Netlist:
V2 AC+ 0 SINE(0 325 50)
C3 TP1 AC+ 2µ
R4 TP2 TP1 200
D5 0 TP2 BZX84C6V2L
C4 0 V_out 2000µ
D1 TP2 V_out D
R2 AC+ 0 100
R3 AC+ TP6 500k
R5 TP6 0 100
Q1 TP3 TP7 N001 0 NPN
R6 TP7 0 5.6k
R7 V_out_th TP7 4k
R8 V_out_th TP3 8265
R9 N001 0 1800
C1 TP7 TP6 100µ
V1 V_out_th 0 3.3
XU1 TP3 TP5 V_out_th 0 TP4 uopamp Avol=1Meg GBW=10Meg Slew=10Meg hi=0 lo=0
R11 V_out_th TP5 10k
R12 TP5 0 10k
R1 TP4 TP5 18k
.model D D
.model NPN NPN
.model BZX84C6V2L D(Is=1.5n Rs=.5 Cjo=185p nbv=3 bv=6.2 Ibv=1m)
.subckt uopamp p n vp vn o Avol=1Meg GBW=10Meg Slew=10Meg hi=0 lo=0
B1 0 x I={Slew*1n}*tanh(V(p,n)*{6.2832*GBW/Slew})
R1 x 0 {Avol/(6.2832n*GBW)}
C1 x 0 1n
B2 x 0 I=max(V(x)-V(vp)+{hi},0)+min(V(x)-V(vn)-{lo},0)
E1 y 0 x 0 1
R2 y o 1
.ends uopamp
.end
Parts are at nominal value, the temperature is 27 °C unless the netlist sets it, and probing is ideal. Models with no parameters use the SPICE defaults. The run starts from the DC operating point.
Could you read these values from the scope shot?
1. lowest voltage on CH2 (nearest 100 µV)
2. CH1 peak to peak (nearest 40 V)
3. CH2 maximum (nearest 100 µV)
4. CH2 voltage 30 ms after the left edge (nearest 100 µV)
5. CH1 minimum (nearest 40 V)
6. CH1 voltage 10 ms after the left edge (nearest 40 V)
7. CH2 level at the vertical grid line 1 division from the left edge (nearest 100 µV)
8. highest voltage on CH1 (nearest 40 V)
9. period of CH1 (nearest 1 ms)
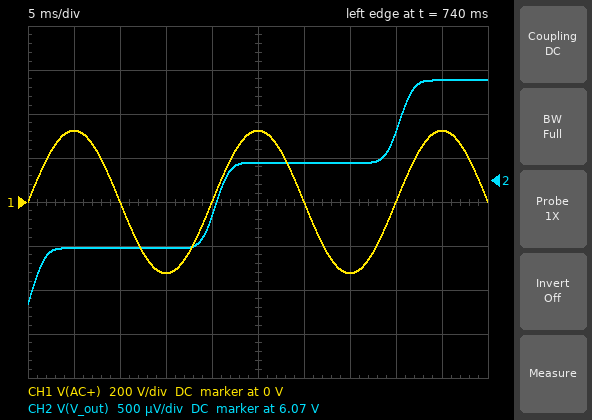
6.0681 V
640 V
6.0706 V
6.0697 V
-320 V
0 V
6.0687 V
320 V
20 ms
